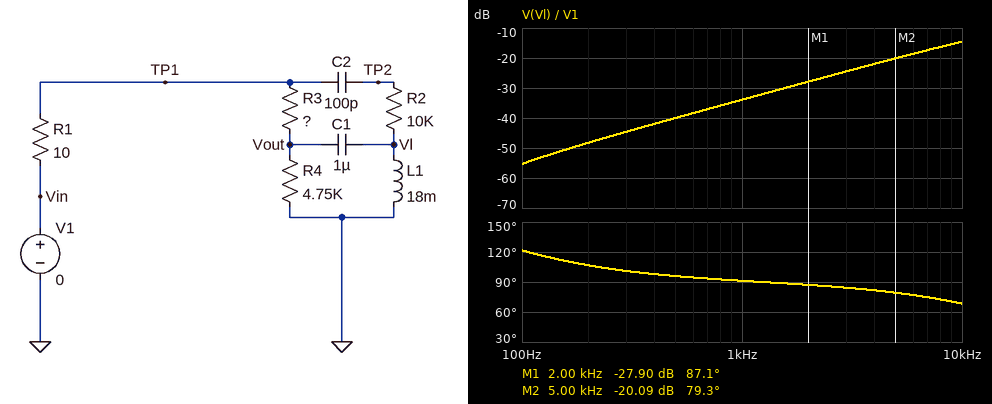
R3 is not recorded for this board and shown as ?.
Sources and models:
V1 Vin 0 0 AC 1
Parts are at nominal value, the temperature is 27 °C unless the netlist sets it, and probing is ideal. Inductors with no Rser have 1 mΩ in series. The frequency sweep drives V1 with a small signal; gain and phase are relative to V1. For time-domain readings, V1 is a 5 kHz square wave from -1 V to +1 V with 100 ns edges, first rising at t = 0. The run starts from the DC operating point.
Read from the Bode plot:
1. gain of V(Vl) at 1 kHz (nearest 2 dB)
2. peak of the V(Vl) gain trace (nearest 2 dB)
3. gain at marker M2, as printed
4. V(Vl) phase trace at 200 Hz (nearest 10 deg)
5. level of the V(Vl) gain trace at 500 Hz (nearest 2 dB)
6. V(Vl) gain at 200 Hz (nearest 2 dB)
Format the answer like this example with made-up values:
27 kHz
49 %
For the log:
-34 dB
-14 dB
-20.09 dB
110 deg
-40 dB
-48 dB
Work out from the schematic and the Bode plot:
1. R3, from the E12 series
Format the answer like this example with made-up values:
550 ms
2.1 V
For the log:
5.6 kΩ
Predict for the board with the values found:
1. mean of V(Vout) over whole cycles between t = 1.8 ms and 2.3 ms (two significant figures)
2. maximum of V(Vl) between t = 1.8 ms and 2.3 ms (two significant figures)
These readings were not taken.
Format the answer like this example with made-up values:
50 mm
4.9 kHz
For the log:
-210 mV
1.1 V
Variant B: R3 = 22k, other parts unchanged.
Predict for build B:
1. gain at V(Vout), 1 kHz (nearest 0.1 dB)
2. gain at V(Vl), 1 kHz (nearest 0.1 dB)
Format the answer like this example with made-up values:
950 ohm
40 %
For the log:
-53.6 dB
-45.8 dB
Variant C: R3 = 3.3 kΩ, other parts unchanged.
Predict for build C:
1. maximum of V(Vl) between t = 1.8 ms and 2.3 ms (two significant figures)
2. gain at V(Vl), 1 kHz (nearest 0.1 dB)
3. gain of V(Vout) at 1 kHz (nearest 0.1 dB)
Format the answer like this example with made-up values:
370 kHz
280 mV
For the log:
1.3 V
-29.3 dB
-37.1 dB
